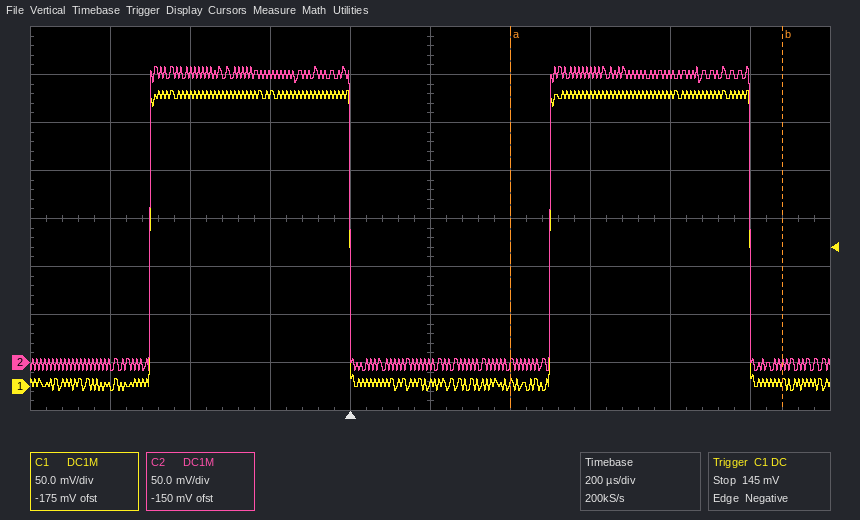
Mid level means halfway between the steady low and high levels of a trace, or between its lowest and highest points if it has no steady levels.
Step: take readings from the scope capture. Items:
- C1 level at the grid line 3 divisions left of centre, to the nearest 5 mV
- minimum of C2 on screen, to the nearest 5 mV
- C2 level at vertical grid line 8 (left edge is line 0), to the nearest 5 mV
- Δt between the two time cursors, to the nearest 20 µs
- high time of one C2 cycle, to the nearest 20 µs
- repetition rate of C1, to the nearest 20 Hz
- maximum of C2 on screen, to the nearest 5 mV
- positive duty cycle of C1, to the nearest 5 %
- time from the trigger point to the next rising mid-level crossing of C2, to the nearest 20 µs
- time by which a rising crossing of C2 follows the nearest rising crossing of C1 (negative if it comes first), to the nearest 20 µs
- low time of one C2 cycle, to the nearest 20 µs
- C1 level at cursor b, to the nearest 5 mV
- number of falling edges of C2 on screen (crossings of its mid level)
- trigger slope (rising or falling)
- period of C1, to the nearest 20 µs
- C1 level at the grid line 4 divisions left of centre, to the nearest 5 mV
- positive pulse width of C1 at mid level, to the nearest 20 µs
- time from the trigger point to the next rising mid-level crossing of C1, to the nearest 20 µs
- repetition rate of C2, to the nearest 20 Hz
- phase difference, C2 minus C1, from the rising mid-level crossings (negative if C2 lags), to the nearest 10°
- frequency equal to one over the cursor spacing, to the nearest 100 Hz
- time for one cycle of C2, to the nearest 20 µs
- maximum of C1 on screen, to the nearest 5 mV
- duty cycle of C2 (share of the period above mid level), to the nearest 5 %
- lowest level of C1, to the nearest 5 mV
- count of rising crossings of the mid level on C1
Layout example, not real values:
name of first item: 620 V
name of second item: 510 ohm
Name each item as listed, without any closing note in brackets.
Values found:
C1 level at the grid line 3 divisions left of centre, to the nearest 5 mV: 305 mV
minimum of C2 on screen, to the nearest 5 mV: -10 mV
C2 level at vertical grid line 8 (left edge is line 0), to the nearest 5 mV: 300 mV
Δt between the two time cursors, to the nearest 20 µs: 680 µs
high time of one C2 cycle, to the nearest 20 µs: 500 µs
repetition rate of C1, to the nearest 20 Hz: 1.00 kHz
maximum of C2 on screen, to the nearest 5 mV: 310 mV
positive duty cycle of C1, to the nearest 5 %: 50 %
time from the trigger point to the next rising mid-level crossing of C2, to the nearest 20 µs: 500 µs
time by which a rising crossing of C2 follows the nearest rising crossing of C1 (negative if it comes first), to the nearest 20 µs: 0 µs
low time of one C2 cycle, to the nearest 20 µs: 500 µs
C1 level at cursor b, to the nearest 5 mV: 5 mV
number of falling edges of C2 on screen: 2
trigger slope: falling
period of C1, to the nearest 20 µs: 1.00 ms
C1 level at the grid line 4 divisions left of centre, to the nearest 5 mV: 0 mV
positive pulse width of C1 at mid level, to the nearest 20 µs: 500 µs
time from the trigger point to the next rising mid-level crossing of C1, to the nearest 20 µs: 500 µs
repetition rate of C2, to the nearest 20 Hz: 1.00 kHz
phase difference, C2 minus C1, from the rising mid-level crossings (negative if C2 lags), to the nearest 10°: 0°
frequency equal to one over the cursor spacing, to the nearest 100 Hz: 1.5 kHz
time for one cycle of C2, to the nearest 20 µs: 1.00 ms
maximum of C1 on screen, to the nearest 5 mV: 310 mV
duty cycle of C2 (share of the period above mid level), to the nearest 5 %: 50 %
lowest level of C1, to the nearest 5 mV: -5 mV
count of rising crossings of the mid level on C1: 2
